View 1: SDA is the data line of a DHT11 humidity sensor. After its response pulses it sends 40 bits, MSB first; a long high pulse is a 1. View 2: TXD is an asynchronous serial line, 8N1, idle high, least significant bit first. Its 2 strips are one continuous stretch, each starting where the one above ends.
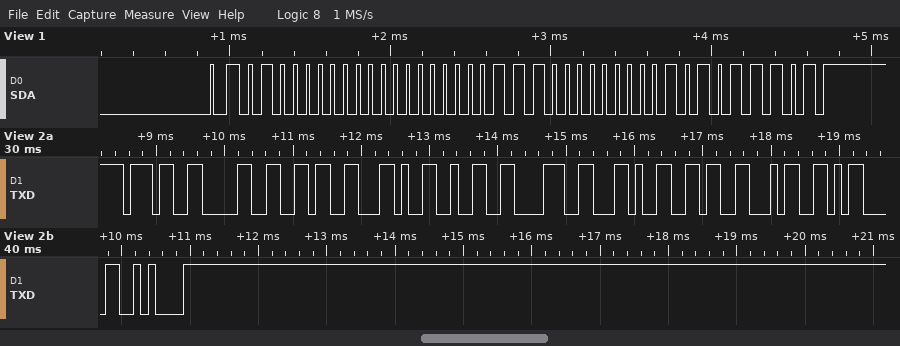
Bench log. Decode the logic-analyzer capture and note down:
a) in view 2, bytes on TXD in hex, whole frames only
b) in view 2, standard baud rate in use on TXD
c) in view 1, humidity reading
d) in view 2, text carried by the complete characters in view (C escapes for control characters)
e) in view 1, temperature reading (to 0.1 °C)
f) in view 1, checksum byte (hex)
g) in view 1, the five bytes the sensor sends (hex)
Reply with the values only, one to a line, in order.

37 30 36 2C 32 38 2C 36 34 0D 0A
9600 baud
64 %
"706,28,64\r\n"
28.1 °C
0x5D
40 00 1C 01 5D
